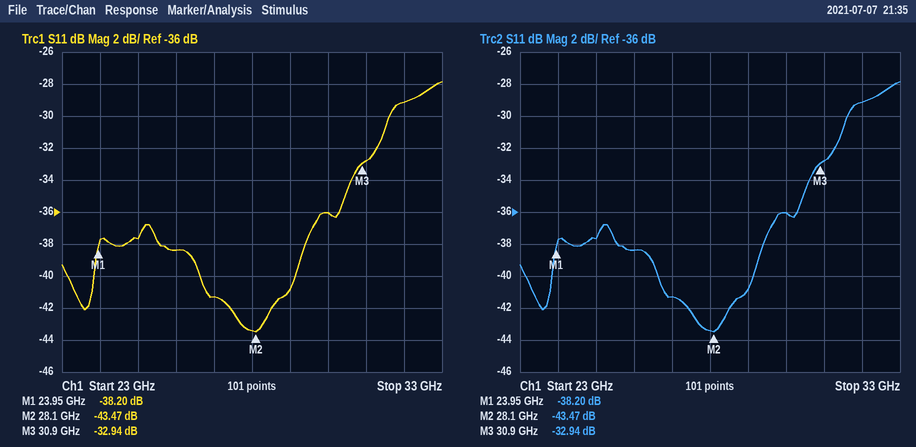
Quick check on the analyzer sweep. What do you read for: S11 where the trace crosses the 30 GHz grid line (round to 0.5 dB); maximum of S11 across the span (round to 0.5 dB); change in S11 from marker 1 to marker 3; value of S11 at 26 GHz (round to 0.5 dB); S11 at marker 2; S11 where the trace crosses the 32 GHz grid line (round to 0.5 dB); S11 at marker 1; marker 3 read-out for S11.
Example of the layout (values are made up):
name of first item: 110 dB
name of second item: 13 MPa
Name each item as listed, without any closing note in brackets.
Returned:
S11 where the trace crosses the 30 GHz grid line: -36.0 dB
maximum of S11 across the span: -28.0 dB
change in S11 from marker 1 to marker 3: 5.26 dB
value of S11 at 26 GHz: -38.5 dB
S11 at marker 2: -43.47 dB
S11 where the trace crosses the 32 GHz grid line: -29.0 dB
S11 at marker 1: -38.20 dB
marker 3 read-out for S11: -32.94 dB
